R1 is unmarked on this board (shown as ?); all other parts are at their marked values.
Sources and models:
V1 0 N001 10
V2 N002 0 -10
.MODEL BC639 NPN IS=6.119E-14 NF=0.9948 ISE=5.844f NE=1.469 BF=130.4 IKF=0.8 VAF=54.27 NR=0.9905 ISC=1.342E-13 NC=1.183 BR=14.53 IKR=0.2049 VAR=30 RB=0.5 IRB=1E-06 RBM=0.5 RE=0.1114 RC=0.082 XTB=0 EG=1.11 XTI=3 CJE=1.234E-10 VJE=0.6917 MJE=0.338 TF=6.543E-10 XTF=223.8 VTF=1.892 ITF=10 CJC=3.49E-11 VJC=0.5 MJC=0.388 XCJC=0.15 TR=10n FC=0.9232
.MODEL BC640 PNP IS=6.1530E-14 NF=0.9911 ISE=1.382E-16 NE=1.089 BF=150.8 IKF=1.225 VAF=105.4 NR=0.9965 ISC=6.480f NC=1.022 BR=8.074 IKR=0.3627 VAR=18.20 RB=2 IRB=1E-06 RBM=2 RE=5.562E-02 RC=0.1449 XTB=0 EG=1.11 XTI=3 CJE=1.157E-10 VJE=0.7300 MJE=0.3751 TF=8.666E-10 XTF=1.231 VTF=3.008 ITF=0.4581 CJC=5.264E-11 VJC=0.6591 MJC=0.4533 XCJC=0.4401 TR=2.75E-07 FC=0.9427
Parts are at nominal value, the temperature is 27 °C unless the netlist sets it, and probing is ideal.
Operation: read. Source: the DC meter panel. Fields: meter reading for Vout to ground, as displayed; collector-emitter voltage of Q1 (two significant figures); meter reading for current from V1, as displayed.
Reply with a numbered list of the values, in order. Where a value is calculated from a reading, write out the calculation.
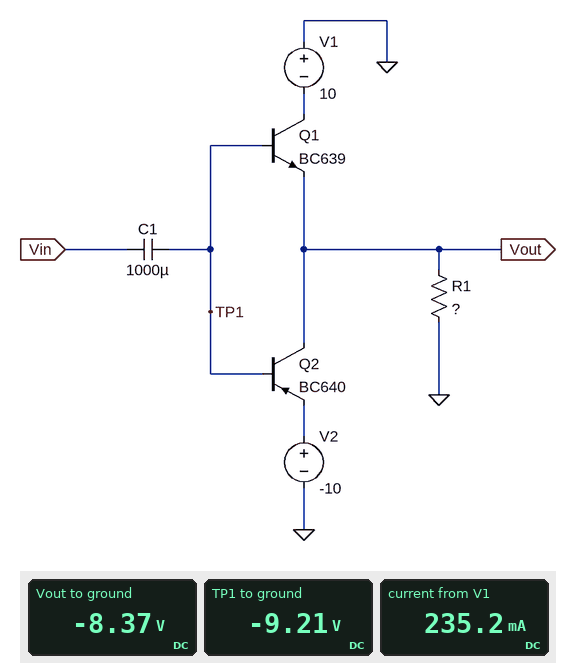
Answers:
1. -8.37 V
2. -10 V - (-8.37 V) = -1.6 V
3. 235.2 mA
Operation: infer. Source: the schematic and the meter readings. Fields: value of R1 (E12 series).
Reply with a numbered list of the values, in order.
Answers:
1. 22 Ω
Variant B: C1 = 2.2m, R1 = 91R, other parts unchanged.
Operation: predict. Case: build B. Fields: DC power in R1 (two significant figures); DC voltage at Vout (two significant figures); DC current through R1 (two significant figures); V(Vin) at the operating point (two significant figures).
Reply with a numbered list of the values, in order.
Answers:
1. 810 mW
2. -8.6 V
3. 94 mA
4. -9.3 V
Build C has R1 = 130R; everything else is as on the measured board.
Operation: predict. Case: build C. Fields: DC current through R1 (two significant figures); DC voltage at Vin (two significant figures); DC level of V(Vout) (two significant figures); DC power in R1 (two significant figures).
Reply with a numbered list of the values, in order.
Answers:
1. 66 mA
2. -9.3 V
3. -8.6 V
4. 570 mW
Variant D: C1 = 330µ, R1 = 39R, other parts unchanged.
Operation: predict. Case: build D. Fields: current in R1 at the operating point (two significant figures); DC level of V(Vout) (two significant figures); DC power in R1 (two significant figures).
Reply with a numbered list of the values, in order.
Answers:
1. 220 mA
2. -8.5 V
3. 1.8 W
